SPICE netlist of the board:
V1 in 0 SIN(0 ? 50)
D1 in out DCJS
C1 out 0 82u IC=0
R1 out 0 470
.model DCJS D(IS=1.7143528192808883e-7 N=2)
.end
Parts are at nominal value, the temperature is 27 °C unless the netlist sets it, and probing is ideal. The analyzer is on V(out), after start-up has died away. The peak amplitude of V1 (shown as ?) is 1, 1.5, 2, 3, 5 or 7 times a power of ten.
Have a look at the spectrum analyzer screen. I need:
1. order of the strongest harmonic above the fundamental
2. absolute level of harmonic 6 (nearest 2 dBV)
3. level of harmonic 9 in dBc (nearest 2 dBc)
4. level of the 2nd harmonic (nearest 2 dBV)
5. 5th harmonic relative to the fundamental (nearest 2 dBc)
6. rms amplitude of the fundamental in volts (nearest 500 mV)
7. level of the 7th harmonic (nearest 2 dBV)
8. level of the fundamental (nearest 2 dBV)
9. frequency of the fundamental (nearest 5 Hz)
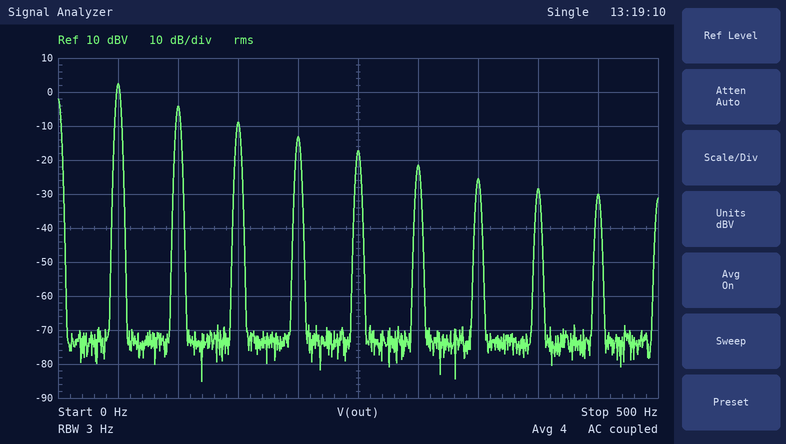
2
-22 dBV
-32 dBc
-4 dBV
-20 dBc
1.5 V
-26 dBV
2 dBV
50 Hz
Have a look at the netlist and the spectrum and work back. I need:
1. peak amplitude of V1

15 V
